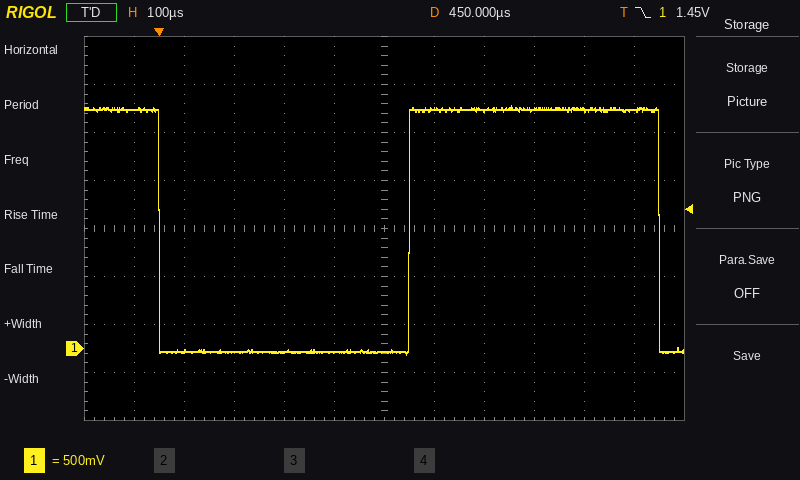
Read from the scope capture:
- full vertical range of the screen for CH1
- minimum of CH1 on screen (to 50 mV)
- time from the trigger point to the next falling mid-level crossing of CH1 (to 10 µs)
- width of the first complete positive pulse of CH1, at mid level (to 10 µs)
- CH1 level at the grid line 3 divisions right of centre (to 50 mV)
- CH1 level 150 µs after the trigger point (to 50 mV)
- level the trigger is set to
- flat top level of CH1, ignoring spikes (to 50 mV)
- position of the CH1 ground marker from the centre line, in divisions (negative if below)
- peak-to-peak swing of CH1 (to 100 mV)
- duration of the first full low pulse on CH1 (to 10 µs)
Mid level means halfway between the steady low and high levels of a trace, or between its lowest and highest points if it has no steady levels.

4 V
-50 mV
1.00 ms
500 µs
2.50 V
-50 mV
1.45 V
2.50 V
-2.5 div
2.60 V
500 µs
